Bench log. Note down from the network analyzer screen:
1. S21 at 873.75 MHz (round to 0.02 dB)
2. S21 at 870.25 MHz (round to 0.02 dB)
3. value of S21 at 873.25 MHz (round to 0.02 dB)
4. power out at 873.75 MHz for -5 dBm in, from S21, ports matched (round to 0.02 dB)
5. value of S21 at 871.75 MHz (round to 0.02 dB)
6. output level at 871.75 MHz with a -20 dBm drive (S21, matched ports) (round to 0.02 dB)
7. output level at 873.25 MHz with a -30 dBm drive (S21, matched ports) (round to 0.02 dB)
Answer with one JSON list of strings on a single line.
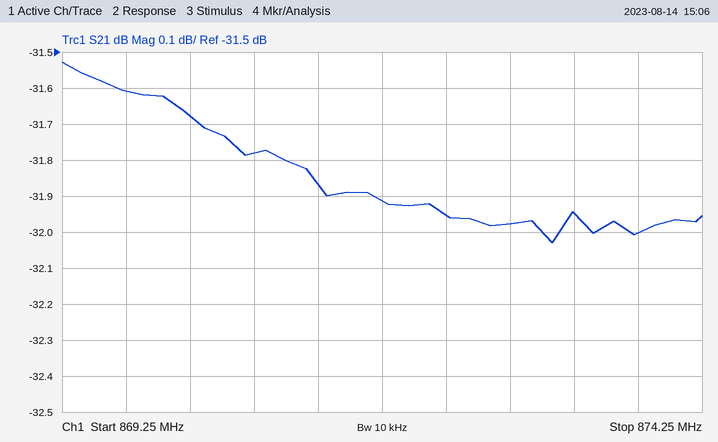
["-32.00 dB", "-31.68 dB", "-31.94 dB", "-37.00 dBm", "-31.92 dB", "-51.92 dBm", "-61.94 dBm"]
